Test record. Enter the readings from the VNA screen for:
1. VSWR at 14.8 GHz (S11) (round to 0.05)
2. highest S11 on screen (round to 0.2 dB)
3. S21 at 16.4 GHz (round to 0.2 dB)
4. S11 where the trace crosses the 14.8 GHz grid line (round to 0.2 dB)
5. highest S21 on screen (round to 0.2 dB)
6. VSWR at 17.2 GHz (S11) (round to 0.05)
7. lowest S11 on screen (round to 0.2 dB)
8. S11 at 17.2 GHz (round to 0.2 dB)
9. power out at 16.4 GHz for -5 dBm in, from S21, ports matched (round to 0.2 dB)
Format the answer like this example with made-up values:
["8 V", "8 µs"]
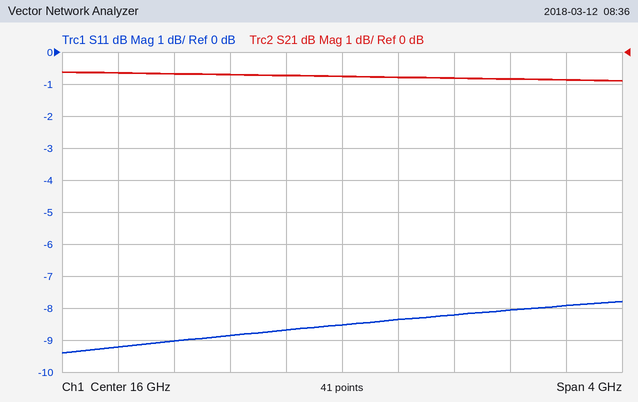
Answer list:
["2.10", "-7.8 dB", "-0.8 dB", "-9.0 dB", "-0.6 dB", "2.30", "-9.4 dB", "-8.0 dB", "-5.8 dBm"]
